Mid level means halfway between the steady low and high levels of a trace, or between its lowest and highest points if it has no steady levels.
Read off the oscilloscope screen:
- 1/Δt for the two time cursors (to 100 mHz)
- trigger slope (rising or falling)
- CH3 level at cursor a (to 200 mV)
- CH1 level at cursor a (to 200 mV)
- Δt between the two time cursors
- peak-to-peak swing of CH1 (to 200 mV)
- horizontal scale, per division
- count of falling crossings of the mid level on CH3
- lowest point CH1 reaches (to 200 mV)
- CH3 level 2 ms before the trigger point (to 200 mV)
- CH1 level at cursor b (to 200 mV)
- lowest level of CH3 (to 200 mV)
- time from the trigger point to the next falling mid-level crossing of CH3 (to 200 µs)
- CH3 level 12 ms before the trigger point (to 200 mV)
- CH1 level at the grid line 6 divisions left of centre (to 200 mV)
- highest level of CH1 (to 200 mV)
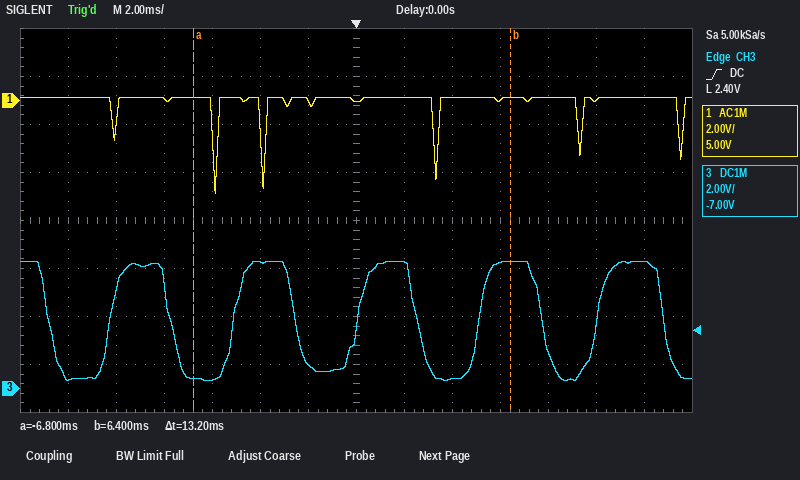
75.8 Hz
rising
400 mV
200 mV
13.2 ms
4.0 V
2 ms
6
-3.8 V
1.0 V
200 mV
400 mV
2.6 ms
400 mV
200 mV
200 mV
